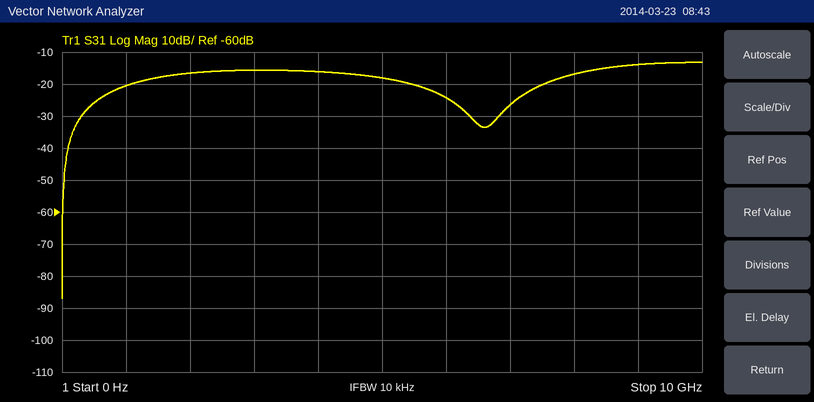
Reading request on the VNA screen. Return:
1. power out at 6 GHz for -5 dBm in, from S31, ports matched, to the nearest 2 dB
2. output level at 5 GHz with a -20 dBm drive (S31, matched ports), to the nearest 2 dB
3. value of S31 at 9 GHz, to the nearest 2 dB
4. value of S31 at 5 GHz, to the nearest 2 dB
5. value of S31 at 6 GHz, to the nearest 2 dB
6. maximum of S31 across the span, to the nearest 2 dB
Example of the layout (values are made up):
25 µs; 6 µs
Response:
-30 dBm; -38 dBm; -14 dB; -18 dB; -24 dB; -14 dB
